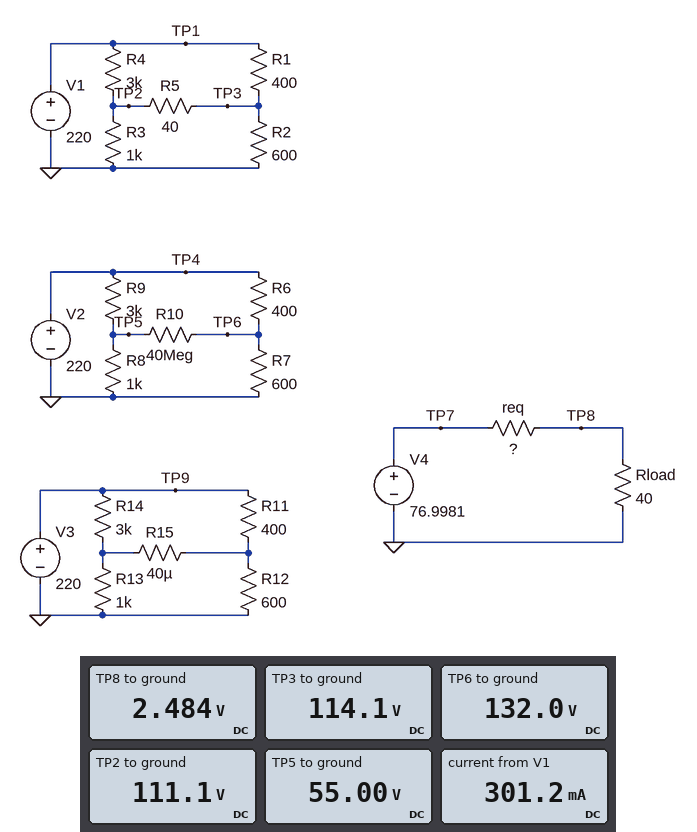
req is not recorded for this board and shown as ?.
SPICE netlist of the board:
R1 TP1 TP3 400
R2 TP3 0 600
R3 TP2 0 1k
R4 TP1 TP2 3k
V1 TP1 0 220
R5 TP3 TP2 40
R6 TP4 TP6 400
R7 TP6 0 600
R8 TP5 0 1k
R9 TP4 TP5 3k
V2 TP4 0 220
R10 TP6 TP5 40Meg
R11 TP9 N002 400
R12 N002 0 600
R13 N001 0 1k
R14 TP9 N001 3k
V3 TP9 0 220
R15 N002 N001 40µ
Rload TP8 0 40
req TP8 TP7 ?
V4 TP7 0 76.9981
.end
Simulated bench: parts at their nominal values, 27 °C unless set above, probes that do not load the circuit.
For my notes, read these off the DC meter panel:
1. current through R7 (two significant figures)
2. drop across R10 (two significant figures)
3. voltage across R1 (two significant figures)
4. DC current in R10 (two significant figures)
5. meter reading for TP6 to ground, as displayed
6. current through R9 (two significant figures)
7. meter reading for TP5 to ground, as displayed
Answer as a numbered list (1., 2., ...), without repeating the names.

1. 220 mA
2. 77 V
3. 110 V
4. 1.9 µA
5. 132.0 V
6. 55 mA
7. 55.00 V
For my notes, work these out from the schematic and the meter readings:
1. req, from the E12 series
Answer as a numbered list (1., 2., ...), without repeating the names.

1. 1.2 kΩ
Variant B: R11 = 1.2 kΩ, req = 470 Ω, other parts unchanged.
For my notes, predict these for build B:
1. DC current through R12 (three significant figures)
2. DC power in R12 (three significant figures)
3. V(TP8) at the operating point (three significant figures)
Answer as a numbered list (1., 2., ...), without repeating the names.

1. 112 mA
2. 7.47 W
3. 6.04 V
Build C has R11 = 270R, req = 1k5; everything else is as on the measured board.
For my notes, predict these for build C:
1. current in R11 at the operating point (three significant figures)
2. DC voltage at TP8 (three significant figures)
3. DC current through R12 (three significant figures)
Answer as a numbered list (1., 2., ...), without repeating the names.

1. 324 mA
2. 2.00 V
3. 221 mA
